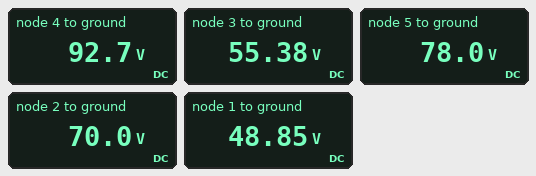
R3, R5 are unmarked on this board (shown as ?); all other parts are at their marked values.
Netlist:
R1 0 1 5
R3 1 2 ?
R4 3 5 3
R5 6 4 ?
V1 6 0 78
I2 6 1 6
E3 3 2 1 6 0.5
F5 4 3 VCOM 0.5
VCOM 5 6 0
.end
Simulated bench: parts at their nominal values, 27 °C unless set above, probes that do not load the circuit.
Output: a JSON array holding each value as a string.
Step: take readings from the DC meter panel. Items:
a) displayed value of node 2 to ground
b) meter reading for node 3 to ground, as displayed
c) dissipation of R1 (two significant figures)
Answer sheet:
["70.0 V", "55.38 V", "480 W"]
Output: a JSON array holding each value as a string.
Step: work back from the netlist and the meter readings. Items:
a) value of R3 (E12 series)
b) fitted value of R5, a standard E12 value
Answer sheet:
["5.6 Ω", "3.9 Ω"]
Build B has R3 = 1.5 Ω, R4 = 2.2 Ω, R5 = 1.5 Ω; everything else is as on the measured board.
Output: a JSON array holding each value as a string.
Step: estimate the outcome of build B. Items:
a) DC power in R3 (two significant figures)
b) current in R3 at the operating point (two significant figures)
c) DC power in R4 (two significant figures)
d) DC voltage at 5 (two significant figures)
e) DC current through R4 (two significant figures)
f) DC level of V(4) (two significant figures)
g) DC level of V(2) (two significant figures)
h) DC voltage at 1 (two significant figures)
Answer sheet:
["43 W", "5.4 A", "250 W", "78 V", "11 A", "86 V", "65 V", "57 V"]
